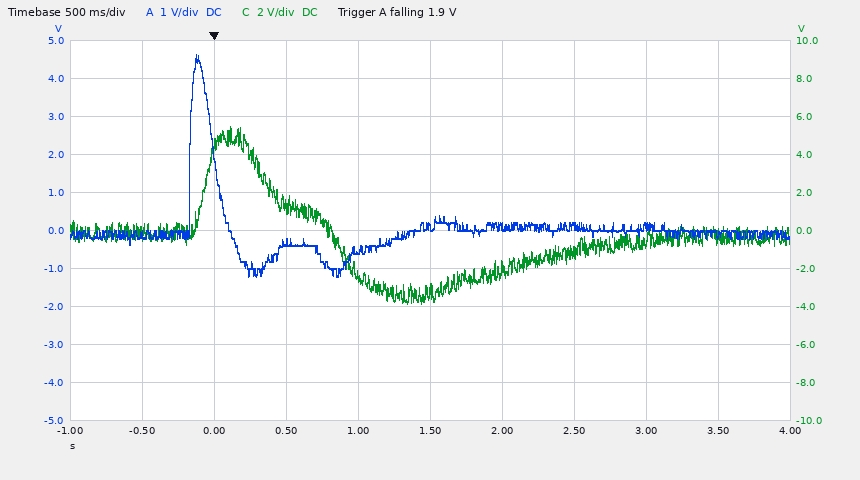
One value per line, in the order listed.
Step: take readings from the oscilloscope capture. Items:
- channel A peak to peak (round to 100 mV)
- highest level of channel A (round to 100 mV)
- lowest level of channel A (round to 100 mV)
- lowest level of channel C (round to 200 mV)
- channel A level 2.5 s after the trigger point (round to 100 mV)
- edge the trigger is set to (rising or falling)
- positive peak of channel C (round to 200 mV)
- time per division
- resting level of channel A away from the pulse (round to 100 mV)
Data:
5.8 V
4.6 V
-1.2 V
-3.8 V
100 mV
falling
5.4 V
500 ms
0.0 V
